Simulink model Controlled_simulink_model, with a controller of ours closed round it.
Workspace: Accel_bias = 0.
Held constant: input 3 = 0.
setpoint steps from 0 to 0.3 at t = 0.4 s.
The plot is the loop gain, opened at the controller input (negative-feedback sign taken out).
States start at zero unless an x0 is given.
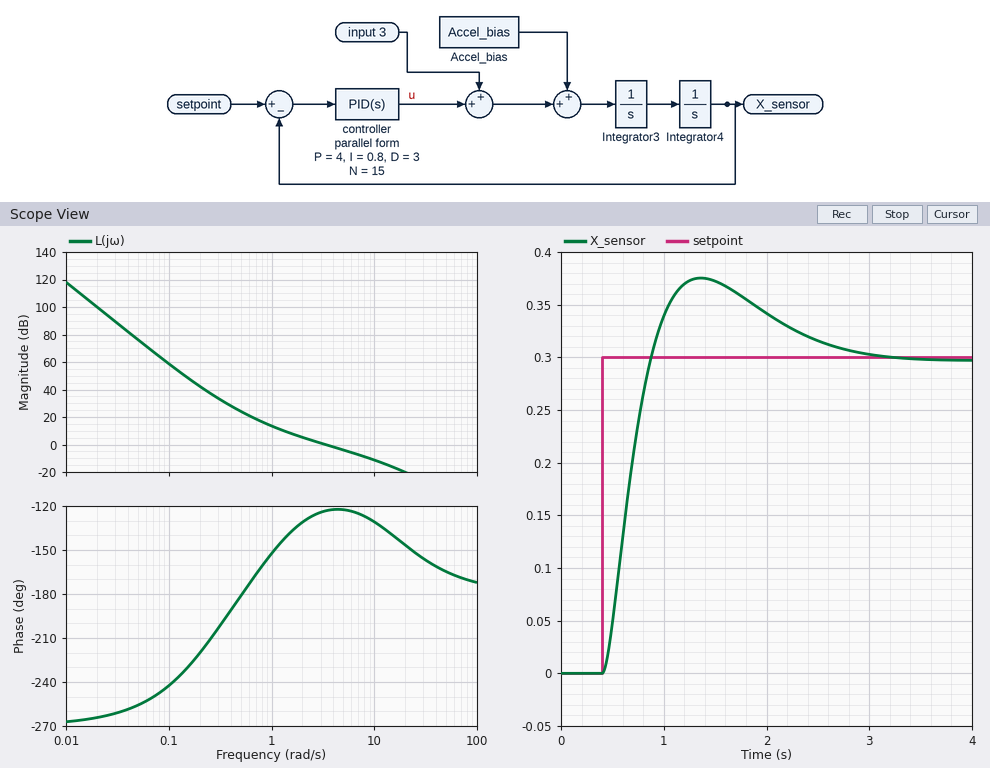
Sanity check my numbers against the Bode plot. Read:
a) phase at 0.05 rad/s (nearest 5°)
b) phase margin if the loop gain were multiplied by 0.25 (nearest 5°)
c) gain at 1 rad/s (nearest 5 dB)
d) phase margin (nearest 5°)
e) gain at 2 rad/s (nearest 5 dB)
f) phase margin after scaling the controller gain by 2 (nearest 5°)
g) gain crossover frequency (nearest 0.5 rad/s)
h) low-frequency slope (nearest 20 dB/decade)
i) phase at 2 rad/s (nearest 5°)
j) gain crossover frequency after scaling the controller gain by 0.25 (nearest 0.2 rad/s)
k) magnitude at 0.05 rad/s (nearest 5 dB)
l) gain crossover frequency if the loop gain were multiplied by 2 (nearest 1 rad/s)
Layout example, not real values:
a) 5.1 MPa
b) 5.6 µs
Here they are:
a) -255°
b) 30°
c) 15 dB
d) 55°
e) 5 dB
f) 55°
g) 3.5 rad/s
h) -60 dB/decade
i) -130°
j) 1.2 rad/s
k) 75 dB
l) 6 rad/s
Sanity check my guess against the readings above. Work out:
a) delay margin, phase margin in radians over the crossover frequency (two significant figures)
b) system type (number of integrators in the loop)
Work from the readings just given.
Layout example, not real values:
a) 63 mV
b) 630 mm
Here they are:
a) 0.27 s
b) 3
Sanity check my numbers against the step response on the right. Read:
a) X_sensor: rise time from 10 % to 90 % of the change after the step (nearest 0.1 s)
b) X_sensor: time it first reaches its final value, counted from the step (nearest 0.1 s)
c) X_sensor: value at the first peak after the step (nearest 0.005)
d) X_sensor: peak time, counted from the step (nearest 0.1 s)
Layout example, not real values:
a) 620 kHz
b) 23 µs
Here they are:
a) 0.3 s
b) 0.5 s
c) 0.375
d) 1.0 s
